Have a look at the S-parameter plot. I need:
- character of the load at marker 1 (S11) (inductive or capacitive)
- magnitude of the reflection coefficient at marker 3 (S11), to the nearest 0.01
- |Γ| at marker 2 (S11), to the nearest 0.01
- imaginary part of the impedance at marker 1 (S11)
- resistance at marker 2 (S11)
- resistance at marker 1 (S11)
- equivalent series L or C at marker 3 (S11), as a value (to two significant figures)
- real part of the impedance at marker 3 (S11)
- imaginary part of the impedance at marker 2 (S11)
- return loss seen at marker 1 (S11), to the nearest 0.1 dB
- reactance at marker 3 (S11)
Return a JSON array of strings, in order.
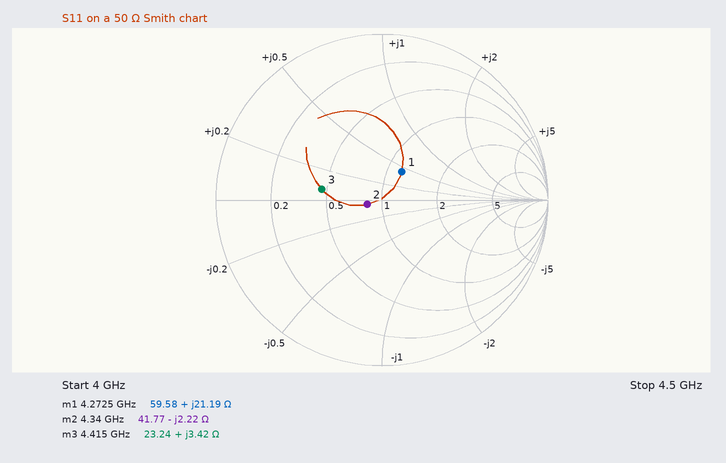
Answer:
["inductive", "0.37", "0.09", "+21.19 Ω", "41.77 Ω", "59.58 Ω", "120 pH", "23.24 Ω", "-2.22 Ω", "13.6 dB", "+3.42 Ω"]
